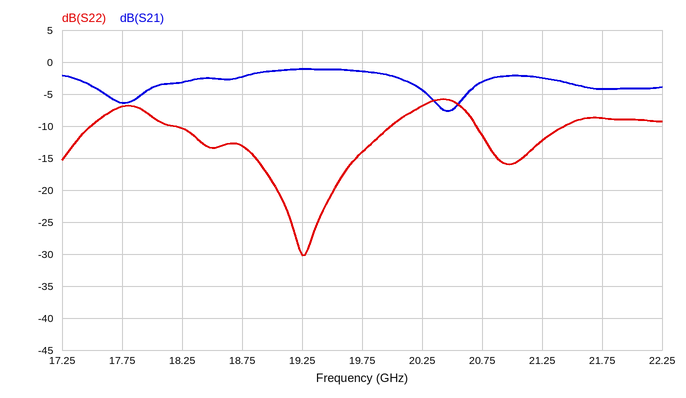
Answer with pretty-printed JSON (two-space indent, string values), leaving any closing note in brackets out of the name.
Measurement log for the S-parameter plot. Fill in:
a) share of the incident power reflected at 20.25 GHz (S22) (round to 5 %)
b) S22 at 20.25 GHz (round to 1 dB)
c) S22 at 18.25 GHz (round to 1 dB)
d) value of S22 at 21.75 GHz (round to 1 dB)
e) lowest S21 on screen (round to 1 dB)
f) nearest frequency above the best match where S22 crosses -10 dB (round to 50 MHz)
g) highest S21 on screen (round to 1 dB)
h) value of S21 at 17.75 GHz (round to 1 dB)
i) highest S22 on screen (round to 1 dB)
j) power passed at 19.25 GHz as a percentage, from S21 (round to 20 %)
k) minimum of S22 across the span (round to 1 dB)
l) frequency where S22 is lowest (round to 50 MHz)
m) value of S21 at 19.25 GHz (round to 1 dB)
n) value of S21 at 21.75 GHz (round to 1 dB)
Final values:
{
  "share of the incident power reflected at 20.25 GHz (S22)": "20 %",
  "S22 at 20.25 GHz": "-7 dB",
  "S22 at 18.25 GHz": "-10 dB",
  "value of S22 at 21.75 GHz": "-9 dB",
  "lowest S21 on screen": "-8 dB",
  "nearest frequency above the best match where S22 crosses -10 dB": "20.00 GHz",
  "highest S21 on screen": "-1 dB",
  "value of S21 at 17.75 GHz": "-6 dB",
  "highest S22 on screen": "-6 dB",
  "power passed at 19.25 GHz as a percentage, from S21": "80 %",
  "minimum of S22 across the span": "-30 dB",
  "frequency where S22 is lowest": "19.25 GHz",
  "value of S21 at 19.25 GHz": "-1 dB",
  "value of S21 at 21.75 GHz": "-4 dB"
}
